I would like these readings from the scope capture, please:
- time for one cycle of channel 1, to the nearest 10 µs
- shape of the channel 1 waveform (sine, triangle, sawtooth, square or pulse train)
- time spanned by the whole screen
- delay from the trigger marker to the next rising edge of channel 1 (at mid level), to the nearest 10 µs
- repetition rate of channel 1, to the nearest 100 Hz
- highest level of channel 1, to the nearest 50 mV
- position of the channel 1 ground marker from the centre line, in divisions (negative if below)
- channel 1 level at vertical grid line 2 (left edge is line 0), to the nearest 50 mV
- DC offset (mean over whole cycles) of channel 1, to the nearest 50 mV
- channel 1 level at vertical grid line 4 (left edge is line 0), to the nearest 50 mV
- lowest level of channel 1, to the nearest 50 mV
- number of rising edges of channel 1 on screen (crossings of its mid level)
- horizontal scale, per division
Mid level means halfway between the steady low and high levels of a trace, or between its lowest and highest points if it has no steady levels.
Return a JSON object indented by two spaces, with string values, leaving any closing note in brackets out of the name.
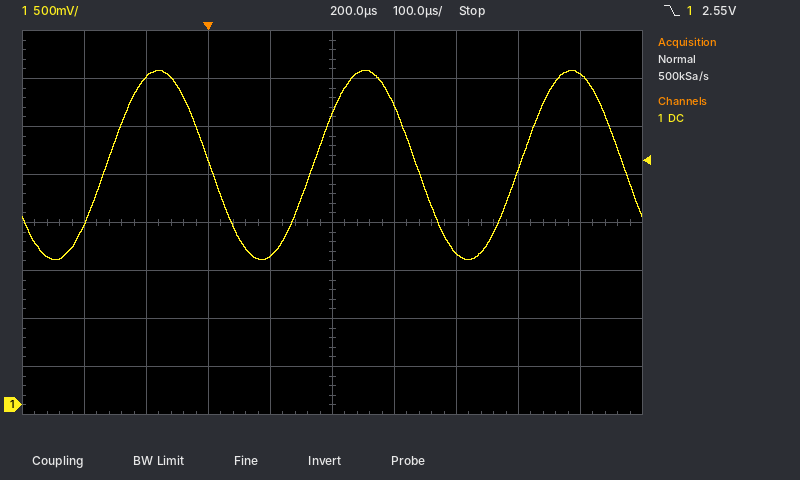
{
  "time for one cycle of channel 1, to the nearest 10 µs": "330 µs",
  "shape of the channel 1 waveform": "sine",
  "time spanned by the whole screen": "1 ms",
  "delay from the trigger marker to the next rising edge of channel 1 (at mid level), to the nearest 10 µs": "170 µs",
  "repetition rate of channel 1, to the nearest 100 Hz": "3.0 kHz",
  "highest level of channel 1, to the nearest 50 mV": "3.50 V",
  "position of the channel 1 ground marker from the centre line, in divisions": "-3.8 div",
  "channel 1 level at vertical grid line 2 (left edge is line 0), to the nearest 50 mV": "3.40 V",
  "DC offset (mean over whole cycles) of channel 1, to the nearest 50 mV": "2.50 V",
  "channel 1 level at vertical grid line 4 (left edge is line 0), to the nearest 50 mV": "1.55 V",
  "lowest level of channel 1, to the nearest 50 mV": "1.50 V",
  "number of rising edges of channel 1 on screen": "3",
  "horizontal scale, per division": "100 µs"
}
